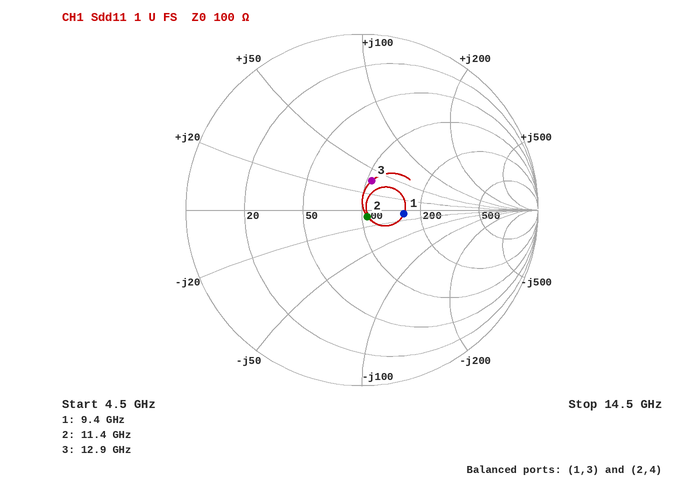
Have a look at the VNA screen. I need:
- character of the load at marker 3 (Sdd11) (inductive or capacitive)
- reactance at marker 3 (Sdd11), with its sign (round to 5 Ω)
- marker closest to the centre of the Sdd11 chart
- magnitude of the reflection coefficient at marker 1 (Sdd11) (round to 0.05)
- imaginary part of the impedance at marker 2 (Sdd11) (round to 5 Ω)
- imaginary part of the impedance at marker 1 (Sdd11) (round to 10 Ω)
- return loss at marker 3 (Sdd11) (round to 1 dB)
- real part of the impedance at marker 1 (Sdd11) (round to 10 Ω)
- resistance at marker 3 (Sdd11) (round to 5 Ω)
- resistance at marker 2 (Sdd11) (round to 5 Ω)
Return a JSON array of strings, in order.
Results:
["inductive", "+35 Ω", "marker 2", "0.25", "-10 Ω", "-10 Ω", "15 dB", "160 Ω", "105 Ω", "105 Ω"]
